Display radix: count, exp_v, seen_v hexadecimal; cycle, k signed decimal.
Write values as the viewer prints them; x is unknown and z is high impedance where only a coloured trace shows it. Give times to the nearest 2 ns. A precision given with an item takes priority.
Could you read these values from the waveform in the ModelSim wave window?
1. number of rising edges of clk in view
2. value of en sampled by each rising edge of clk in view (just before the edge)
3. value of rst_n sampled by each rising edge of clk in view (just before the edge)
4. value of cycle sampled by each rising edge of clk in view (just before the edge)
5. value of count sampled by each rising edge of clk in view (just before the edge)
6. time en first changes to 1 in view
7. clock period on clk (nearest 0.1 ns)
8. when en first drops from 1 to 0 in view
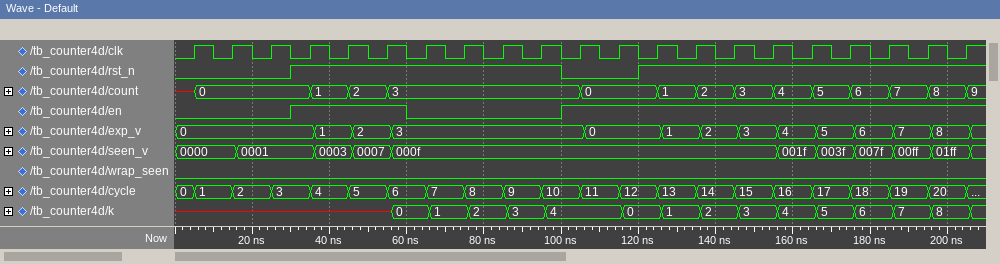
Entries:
21
0 0 0 1 1 1 0 0 0 0 1 1 1 1 1 1 1 1 1 1 1
0 0 0 1 1 1 1 1 1 1 0 0 1 1 1 1 1 1 1 1 1
0, 1, 2, 3, 4, 5, 6, 7, 8, 9, 10, 11, 12, 13, 14, 15, 16, 17, 18, 19, 20
x, 0, 0, 0, 1, 2, 3, 3, 3, 3, 3, 0, 0, 1, 2, 3, 4, 5, 6, 7, 8
30 ns
10 ns
60 ns
